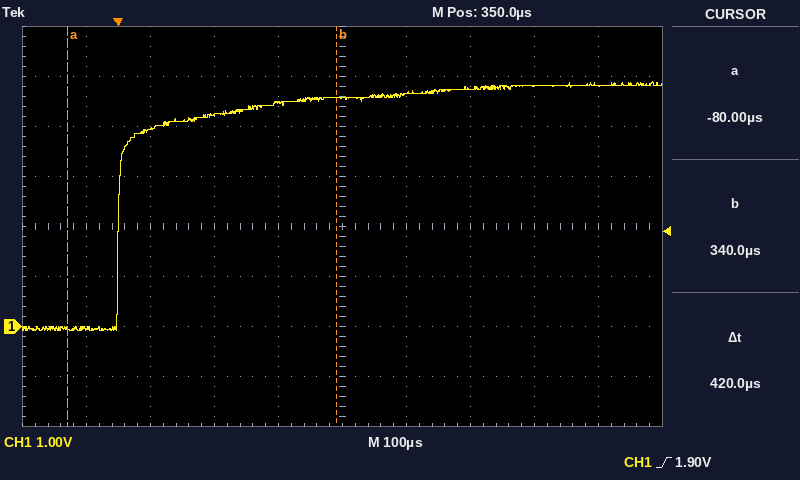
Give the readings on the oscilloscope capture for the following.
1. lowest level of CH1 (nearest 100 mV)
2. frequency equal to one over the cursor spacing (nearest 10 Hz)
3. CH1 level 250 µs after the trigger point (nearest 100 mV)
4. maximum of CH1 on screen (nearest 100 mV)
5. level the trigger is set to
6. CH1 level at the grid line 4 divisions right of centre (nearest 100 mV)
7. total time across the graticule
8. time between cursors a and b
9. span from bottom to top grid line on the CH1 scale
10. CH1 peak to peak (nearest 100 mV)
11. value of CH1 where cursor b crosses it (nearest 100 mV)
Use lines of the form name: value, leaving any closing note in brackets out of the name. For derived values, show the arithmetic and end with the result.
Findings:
lowest level of CH1: -100 mV
frequency equal to one over the cursor spacing: 1 / 420 µs ≈ 2.38 kHz
CH1 level 250 µs after the trigger point: 4.5 V
maximum of CH1 on screen: 4.9 V
level the trigger is set to: 1.90 V
CH1 level at the grid line 4 divisions right of centre: 4.8 V
total time across the graticule: 1 ms
time between cursors a and b: 420 µs
span from bottom to top grid line on the CH1 scale: 8 V
CH1 peak to peak: 4.9 V − (-100 mV) = 5.0 V
value of CH1 where cursor b crosses it: 4.6 V
